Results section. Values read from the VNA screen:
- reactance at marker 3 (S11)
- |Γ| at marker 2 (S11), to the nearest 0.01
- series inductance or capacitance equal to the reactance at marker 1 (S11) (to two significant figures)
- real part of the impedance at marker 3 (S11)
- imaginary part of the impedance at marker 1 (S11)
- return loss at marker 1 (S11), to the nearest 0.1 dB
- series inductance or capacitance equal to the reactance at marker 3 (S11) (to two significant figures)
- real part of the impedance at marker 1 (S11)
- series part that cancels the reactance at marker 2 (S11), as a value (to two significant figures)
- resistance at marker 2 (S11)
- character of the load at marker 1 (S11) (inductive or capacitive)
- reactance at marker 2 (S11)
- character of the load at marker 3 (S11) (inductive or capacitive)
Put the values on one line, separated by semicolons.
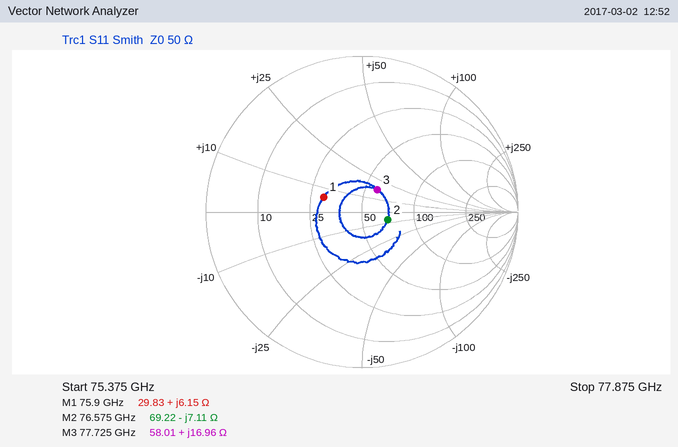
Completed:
+16.96 Ω; 0.17; 13 pH; 58.01 Ω; +6.15 Ω; 11.6 dB; 35 pH; 29.83 Ω; 15 pH; 69.22 Ω; inductive; -7.11 Ω; inductive
